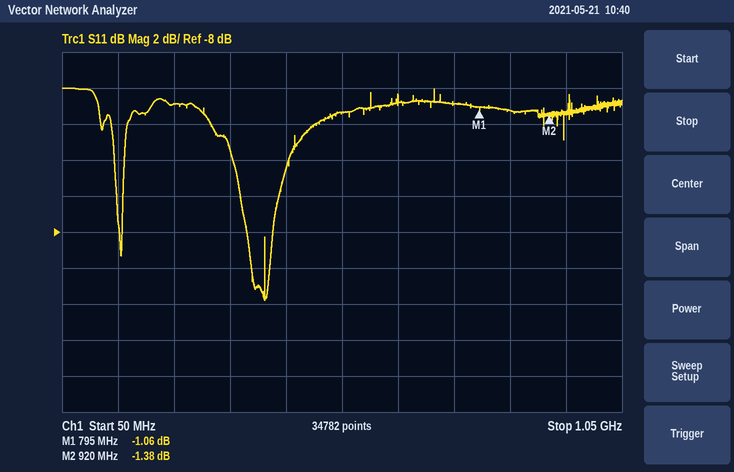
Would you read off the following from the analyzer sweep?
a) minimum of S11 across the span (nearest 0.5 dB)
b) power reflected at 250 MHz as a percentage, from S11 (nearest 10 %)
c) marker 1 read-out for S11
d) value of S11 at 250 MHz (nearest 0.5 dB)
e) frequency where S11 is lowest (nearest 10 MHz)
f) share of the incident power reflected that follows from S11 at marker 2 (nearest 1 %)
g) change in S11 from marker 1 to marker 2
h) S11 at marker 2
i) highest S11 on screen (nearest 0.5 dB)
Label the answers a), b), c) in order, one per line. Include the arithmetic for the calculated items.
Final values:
a) -12.0 dB
b) 10^(-1/10) ≈ 79.4 %, so 80 % to the nearest 10 %
c) -1.06 dB
d) -1.0 dB
e) 410 MHz
f) 10^(-1.38/10) ≈ 73 %
g) -1.38 − (-1.06) = -0.32 dB
h) -1.38 dB
i) 0.0 dB
